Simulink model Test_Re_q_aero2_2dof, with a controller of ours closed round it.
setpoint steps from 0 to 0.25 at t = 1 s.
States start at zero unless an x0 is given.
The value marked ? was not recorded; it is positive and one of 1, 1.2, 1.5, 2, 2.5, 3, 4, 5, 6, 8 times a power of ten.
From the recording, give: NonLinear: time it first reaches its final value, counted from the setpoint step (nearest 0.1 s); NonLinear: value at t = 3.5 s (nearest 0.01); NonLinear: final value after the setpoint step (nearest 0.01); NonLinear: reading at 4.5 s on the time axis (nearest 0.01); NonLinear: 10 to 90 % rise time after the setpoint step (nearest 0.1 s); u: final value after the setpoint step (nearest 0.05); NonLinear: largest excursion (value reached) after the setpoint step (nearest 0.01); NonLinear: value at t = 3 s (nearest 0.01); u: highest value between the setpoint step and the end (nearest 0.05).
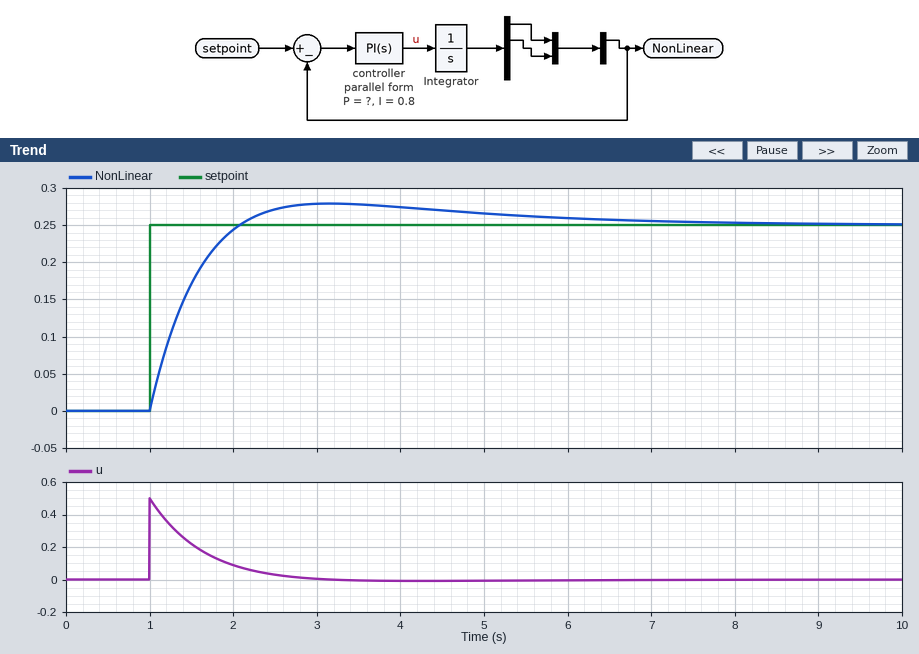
1.1 s
0.28
0.25
0.27
0.8 s
0.00
0.28
0.28
0.50
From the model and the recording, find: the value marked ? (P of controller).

2
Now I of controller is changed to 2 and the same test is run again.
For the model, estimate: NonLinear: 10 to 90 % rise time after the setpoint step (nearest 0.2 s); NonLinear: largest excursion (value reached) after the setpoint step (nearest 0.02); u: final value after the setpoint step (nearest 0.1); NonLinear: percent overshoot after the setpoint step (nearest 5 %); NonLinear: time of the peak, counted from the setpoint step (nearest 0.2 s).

0.6 s
0.30
0.0
20 %
1.6 s
